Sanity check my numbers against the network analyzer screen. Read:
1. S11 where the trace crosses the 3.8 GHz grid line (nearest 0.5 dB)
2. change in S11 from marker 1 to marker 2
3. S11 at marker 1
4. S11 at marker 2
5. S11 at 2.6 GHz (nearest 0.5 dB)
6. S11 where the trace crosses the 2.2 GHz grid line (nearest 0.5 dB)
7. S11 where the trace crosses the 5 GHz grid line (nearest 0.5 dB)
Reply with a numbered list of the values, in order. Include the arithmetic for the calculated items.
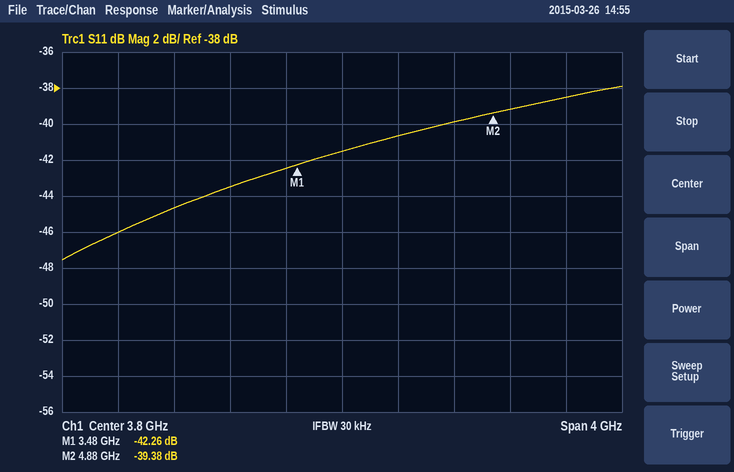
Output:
1. -41.5 dB
2. -39.38 − (-42.26) = 2.88 dB
3. -42.26 dB
4. -39.38 dB
5. -44.5 dB
6. -46.0 dB
7. -39.0 dB
